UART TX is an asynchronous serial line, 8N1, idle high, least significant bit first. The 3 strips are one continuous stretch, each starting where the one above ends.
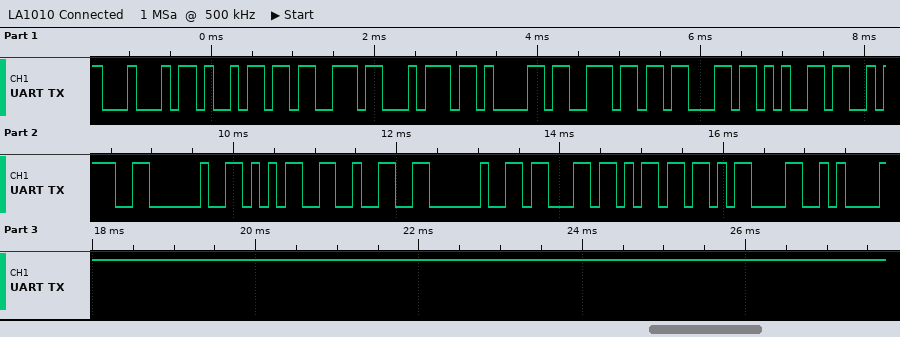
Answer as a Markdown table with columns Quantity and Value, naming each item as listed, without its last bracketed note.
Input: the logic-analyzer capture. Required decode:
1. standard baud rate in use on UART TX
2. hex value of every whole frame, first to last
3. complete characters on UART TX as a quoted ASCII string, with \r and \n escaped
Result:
| Quantity | Value |
|---|---|
| standard baud rate in use on UART TX | 9600 baud |
| hex value of every whole frame, first to last | 44 69 73 74 61 6E 63 65 3A 20 35 32 20 63 6D 0D 0A |
| complete characters on UART TX as a quoted ASCII string, with \r and \n escaped | "Distance: 52 cm\r\n" |
